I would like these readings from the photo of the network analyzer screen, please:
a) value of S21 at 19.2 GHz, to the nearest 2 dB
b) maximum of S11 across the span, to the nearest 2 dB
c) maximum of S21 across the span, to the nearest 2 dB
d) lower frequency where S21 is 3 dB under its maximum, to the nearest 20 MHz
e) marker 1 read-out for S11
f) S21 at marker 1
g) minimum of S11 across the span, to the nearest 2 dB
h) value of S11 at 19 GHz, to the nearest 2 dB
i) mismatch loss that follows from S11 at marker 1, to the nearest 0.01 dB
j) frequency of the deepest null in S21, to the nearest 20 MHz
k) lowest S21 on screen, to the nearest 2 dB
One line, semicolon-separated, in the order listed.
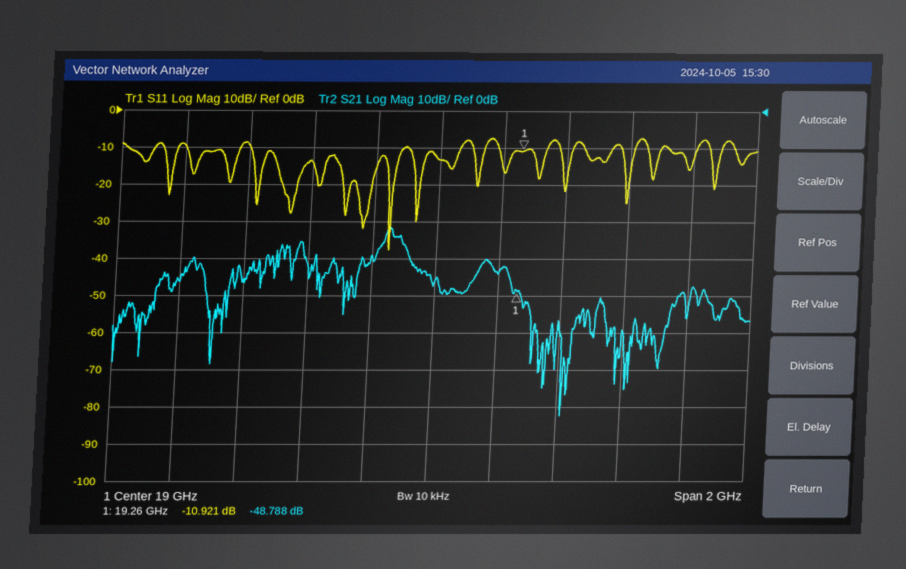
-44 dB; -8 dB; -32 dB; 18.84 GHz; -10.921 dB; -48.788 dB; -38 dB; -14 dB; 0.37 dB; 19.42 GHz; -82 dB
